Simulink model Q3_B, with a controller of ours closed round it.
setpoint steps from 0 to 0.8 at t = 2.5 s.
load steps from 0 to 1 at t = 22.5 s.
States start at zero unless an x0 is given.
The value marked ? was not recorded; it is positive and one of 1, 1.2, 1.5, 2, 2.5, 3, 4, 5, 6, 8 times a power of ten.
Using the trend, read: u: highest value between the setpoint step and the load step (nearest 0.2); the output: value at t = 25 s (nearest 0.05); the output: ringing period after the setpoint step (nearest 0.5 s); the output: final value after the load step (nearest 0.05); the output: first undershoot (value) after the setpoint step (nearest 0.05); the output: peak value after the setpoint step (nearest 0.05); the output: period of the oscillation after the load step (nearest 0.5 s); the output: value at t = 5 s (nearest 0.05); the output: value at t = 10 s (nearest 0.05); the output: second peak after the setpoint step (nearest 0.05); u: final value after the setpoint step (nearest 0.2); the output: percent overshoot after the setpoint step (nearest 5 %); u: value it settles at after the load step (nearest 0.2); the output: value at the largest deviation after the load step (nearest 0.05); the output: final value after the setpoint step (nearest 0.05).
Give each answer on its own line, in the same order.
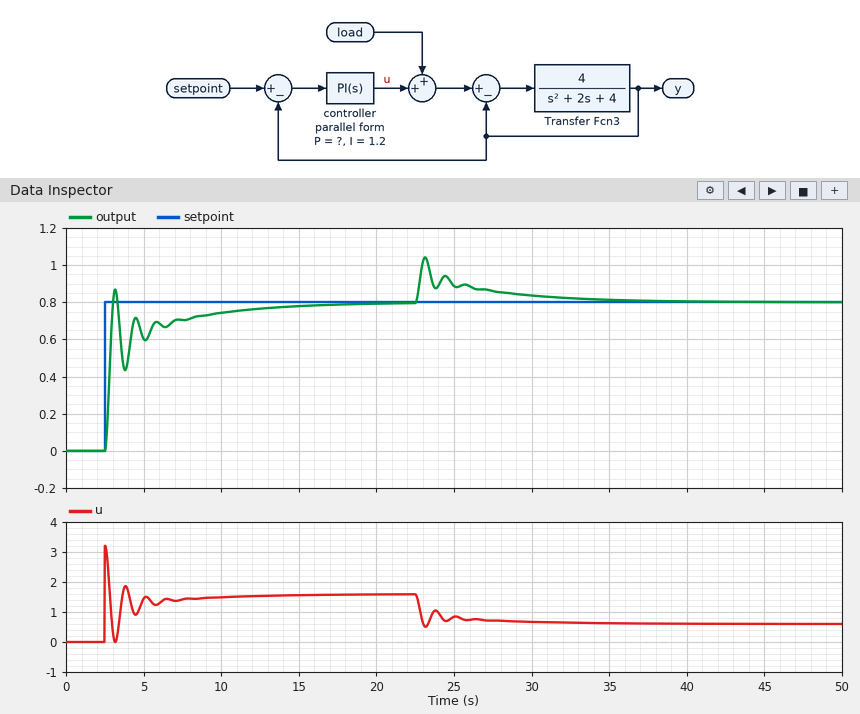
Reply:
3.2
0.90
1.5 s
0.80
0.45
0.85
1.5 s
0.60
0.75
0.70
1.6
10 %
0.6
1.05
0.80
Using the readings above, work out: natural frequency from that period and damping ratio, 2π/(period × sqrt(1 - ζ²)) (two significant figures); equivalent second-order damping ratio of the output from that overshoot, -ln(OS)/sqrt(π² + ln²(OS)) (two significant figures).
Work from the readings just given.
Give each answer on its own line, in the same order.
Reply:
5.2 rad/s
0.59
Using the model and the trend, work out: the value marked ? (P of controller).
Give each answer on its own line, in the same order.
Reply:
4
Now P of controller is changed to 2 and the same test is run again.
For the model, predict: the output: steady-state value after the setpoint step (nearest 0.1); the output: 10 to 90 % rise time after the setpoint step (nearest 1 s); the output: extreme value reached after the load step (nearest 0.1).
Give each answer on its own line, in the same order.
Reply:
0.8
5 s
1.1
